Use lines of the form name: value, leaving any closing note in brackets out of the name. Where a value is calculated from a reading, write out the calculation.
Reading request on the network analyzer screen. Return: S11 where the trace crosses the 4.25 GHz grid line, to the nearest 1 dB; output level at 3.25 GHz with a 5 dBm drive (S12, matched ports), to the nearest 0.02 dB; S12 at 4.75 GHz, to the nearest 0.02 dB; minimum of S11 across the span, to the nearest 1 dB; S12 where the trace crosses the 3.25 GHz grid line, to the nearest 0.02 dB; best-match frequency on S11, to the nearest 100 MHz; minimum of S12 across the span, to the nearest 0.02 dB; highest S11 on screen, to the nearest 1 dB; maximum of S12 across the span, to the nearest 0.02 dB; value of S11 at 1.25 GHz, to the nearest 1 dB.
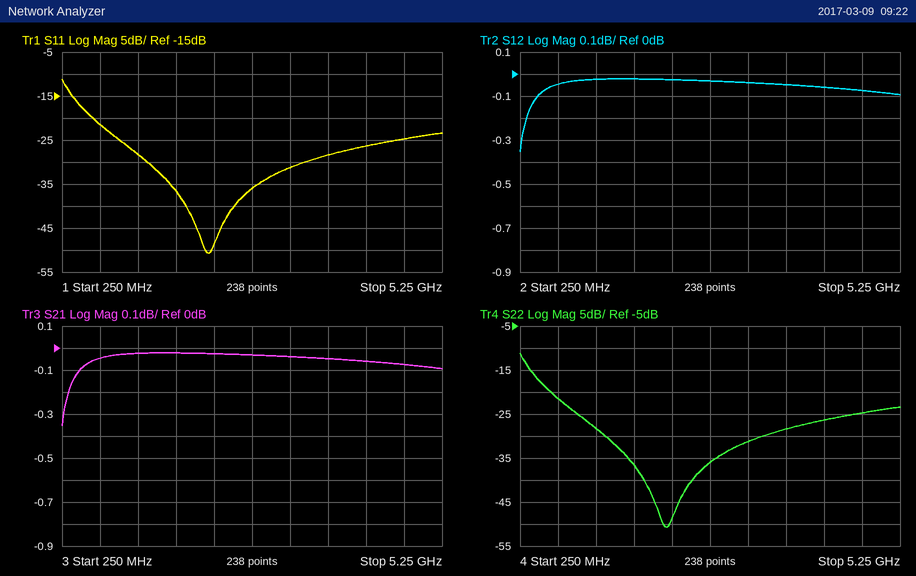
S11 where the trace crosses the 4.25 GHz grid line, to the nearest 1 dB: -26 dB
output level at 3.25 GHz with a 5 dBm drive (S12, matched ports), to the nearest 0.02 dB: 5 dBm + (-0.04 dB) = 4.96 dBm
S12 at 4.75 GHz, to the nearest 0.02 dB: -0.08 dB
minimum of S11 across the span, to the nearest 1 dB: -51 dB
S12 where the trace crosses the 3.25 GHz grid line, to the nearest 0.02 dB: -0.04 dB
best-match frequency on S11, to the nearest 100 MHz: 2.2 GHz
minimum of S12 across the span, to the nearest 0.02 dB: -0.36 dB
highest S11 on screen, to the nearest 1 dB: -11 dB
maximum of S12 across the span, to the nearest 0.02 dB: -0.02 dB
value of S11 at 1.25 GHz, to the nearest 1 dB: -28 dB
